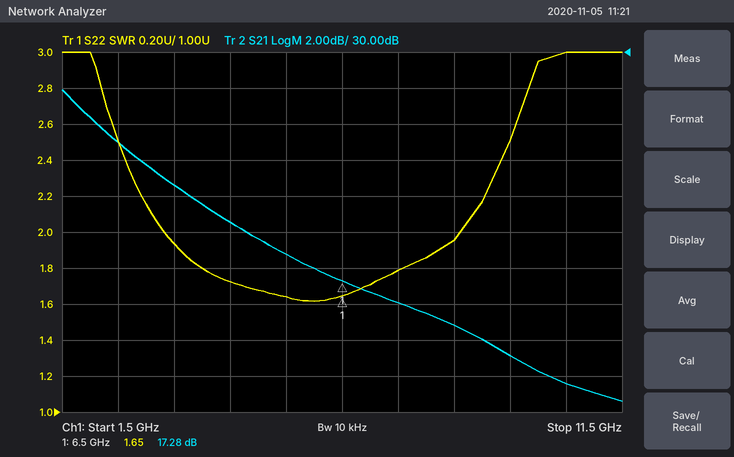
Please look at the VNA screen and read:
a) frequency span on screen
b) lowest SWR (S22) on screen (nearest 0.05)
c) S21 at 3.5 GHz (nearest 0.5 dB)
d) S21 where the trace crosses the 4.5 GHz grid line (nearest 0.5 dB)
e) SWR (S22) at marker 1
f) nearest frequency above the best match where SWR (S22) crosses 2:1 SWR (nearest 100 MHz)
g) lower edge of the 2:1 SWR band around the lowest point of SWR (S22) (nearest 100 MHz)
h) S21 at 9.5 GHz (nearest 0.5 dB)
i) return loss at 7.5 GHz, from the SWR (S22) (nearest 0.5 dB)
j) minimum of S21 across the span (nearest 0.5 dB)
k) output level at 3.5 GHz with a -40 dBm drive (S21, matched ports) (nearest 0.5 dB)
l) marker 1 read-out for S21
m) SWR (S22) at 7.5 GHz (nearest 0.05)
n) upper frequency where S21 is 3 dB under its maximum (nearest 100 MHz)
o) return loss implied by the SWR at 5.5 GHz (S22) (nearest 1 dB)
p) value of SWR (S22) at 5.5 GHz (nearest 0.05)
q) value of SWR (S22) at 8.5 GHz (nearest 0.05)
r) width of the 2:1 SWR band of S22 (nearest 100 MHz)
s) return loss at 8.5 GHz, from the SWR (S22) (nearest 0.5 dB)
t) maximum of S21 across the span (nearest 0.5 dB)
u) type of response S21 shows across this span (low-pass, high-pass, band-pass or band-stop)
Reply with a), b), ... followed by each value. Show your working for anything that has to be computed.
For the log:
a) 10 GHz
b) 1.60
c) 22.5 dB
d) 20.5 dB
e) 1.65
f) 8.6 GHz
g) 3.3 GHz
h) 13.0 dB
i) −20 log10((1.8 − 1)/(1.8 + 1)) ≈ 10.9 dB, so 11.0 dB to the nearest 0.5 dB
j) 10.5 dB
k) -40 dBm + (22.5 dB) = -17.5 dBm
l) 17.28 dB
m) 1.80
n) 2.5 GHz
o) −20 log10((1.65 − 1)/(1.65 + 1)) ≈ 12 dB
p) 1.65
q) 1.95
r) 8.6 GHz − 3.3 GHz = 5.3 GHz
s) −20 log10((1.95 − 1)/(1.95 + 1)) ≈ 9.84 dB, so 10.0 dB to the nearest 0.5 dB
t) 28.0 dB
u) low-pass
